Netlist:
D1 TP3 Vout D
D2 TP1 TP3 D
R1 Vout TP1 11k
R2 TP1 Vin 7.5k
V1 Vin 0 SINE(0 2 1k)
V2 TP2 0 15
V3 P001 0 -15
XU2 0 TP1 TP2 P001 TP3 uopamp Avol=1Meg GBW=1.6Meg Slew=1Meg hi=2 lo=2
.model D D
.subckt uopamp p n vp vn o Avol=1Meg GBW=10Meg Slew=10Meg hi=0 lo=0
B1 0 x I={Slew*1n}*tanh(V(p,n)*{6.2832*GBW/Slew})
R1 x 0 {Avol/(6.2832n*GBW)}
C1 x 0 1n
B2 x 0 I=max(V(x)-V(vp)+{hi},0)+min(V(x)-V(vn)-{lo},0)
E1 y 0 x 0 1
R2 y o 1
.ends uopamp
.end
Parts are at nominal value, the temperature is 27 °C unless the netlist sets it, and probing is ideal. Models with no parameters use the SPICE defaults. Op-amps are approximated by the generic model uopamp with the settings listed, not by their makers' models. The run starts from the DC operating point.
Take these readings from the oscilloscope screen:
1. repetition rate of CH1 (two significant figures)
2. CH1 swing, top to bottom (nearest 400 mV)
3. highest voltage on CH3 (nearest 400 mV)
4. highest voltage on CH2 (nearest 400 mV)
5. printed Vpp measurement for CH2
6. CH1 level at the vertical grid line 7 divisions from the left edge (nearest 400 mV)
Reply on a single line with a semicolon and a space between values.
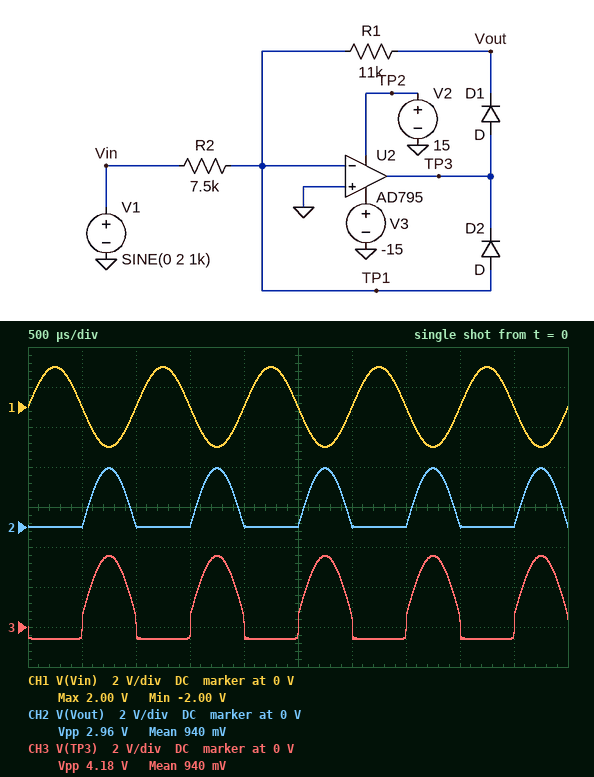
1.0 kHz; 4.0 V; 3.6 V; 2.8 V; 2.96 V; 0 V
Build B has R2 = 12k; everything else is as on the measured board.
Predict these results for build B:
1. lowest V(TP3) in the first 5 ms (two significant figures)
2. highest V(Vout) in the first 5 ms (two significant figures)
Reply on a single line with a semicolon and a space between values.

-610 mV; 1.8 V
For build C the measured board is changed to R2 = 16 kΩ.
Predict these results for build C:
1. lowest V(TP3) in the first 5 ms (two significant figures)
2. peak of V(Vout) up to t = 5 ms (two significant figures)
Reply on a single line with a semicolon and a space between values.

-600 mV; 1.4 V
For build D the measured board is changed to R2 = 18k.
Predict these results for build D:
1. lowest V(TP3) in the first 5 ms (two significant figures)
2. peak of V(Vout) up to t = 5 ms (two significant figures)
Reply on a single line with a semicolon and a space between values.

-600 mV; 1.2 V
